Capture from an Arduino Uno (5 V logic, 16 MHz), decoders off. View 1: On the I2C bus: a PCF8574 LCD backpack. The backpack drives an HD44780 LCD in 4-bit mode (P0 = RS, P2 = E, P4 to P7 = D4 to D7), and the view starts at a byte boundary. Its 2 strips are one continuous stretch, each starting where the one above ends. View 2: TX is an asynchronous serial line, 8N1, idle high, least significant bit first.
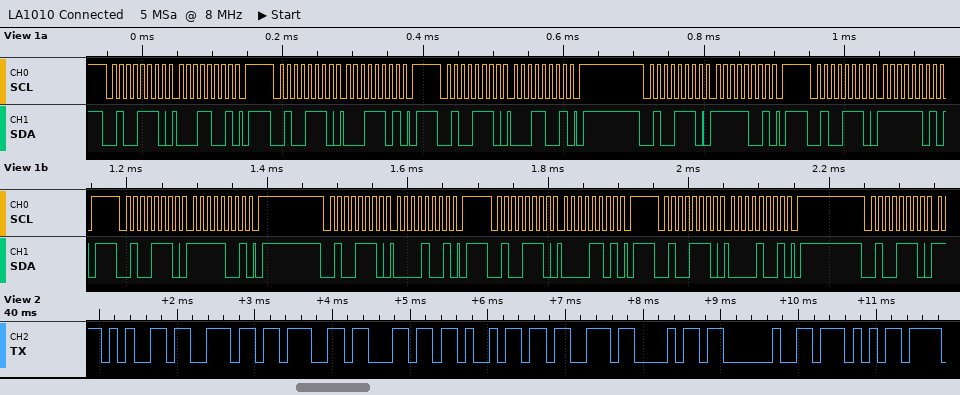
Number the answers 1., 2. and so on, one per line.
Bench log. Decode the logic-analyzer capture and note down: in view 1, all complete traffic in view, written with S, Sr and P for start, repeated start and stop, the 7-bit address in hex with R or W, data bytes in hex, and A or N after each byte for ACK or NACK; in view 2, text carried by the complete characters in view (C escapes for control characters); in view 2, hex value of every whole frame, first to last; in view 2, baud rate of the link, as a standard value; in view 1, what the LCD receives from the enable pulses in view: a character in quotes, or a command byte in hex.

1. S 27W A 19 A P S 27W A 1D A P S 27W A 19 A P S 27W A F9 A P S 27W A FD A P S 27W A F9 A P S 27W A 09 A P S 27W A 0D A P S 27W A 09 A P S 27W A
2. "english W"
3. 65 6E 67 6C 69 73 68 20 57
4. 9600 baud
5. data 0x1F
